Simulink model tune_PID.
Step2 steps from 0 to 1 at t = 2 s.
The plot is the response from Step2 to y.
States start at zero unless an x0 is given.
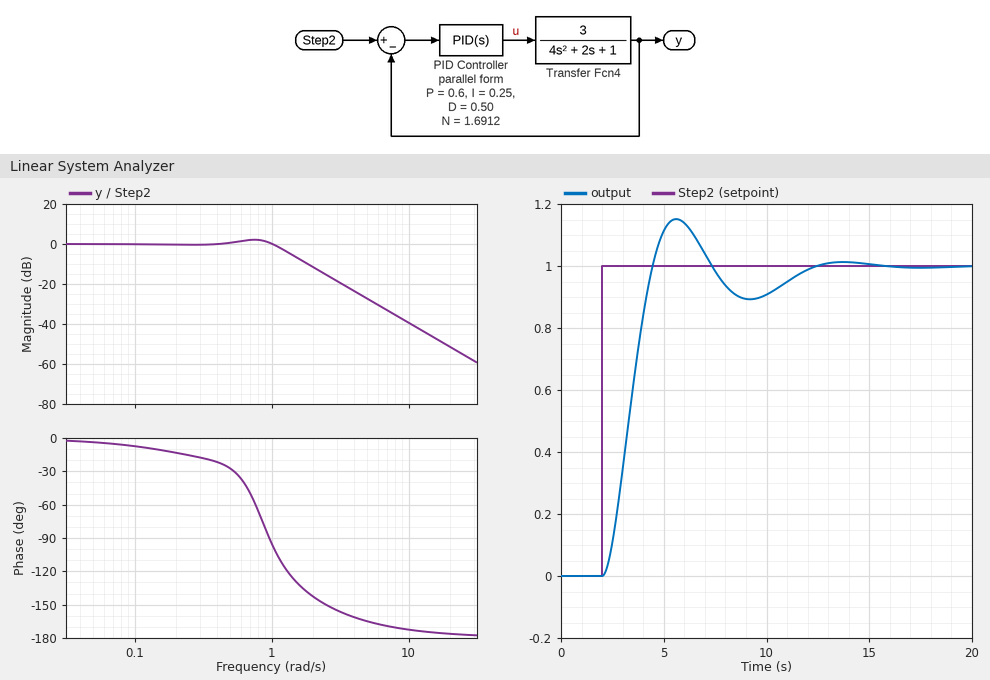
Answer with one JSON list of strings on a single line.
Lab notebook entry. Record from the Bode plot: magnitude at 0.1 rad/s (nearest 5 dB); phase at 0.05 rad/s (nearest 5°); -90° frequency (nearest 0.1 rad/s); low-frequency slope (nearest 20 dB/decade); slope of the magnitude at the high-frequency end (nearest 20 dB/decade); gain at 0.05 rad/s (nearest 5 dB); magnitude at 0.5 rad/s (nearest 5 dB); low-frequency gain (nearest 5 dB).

["0 dB", "-5°", "1.0 rad/s", "0 dB/decade", "-40 dB/decade", "0 dB", "0 dB", "0 dB"]
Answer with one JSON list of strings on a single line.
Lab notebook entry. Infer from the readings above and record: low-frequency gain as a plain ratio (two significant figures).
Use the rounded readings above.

["1.0"]
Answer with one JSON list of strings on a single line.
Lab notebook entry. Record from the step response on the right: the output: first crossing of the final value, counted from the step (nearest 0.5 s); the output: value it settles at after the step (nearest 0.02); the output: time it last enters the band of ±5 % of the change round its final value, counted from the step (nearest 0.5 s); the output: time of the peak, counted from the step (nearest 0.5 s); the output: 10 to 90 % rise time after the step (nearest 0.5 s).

["2.5 s", "1.00", "9.0 s", "3.5 s", "1.5 s"]
